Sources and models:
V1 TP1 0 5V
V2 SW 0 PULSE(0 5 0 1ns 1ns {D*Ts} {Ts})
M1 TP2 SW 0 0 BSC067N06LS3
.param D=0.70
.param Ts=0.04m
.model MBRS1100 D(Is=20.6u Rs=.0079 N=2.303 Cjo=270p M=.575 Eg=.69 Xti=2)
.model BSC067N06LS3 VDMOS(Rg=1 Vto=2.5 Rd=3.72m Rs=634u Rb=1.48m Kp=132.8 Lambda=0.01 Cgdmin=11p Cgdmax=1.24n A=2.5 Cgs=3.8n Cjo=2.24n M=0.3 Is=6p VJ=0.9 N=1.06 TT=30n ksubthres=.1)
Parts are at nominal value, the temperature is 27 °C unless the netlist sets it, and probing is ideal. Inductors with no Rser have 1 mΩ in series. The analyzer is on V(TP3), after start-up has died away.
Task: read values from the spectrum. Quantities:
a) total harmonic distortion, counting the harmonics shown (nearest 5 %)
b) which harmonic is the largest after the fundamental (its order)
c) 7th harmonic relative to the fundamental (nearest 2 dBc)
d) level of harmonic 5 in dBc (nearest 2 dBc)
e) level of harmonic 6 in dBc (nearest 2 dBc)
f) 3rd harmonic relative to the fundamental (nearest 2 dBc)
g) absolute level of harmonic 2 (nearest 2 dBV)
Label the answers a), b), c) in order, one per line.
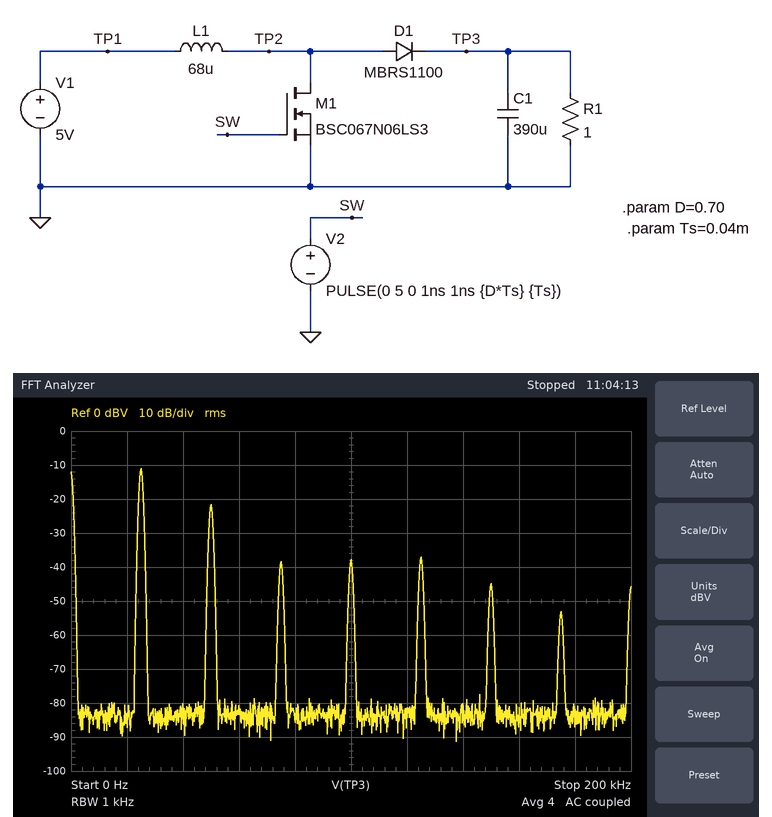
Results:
a) 30 %
b) 2
c) -42 dBc
d) -26 dBc
e) -34 dBc
f) -28 dBc
g) -22 dBV
